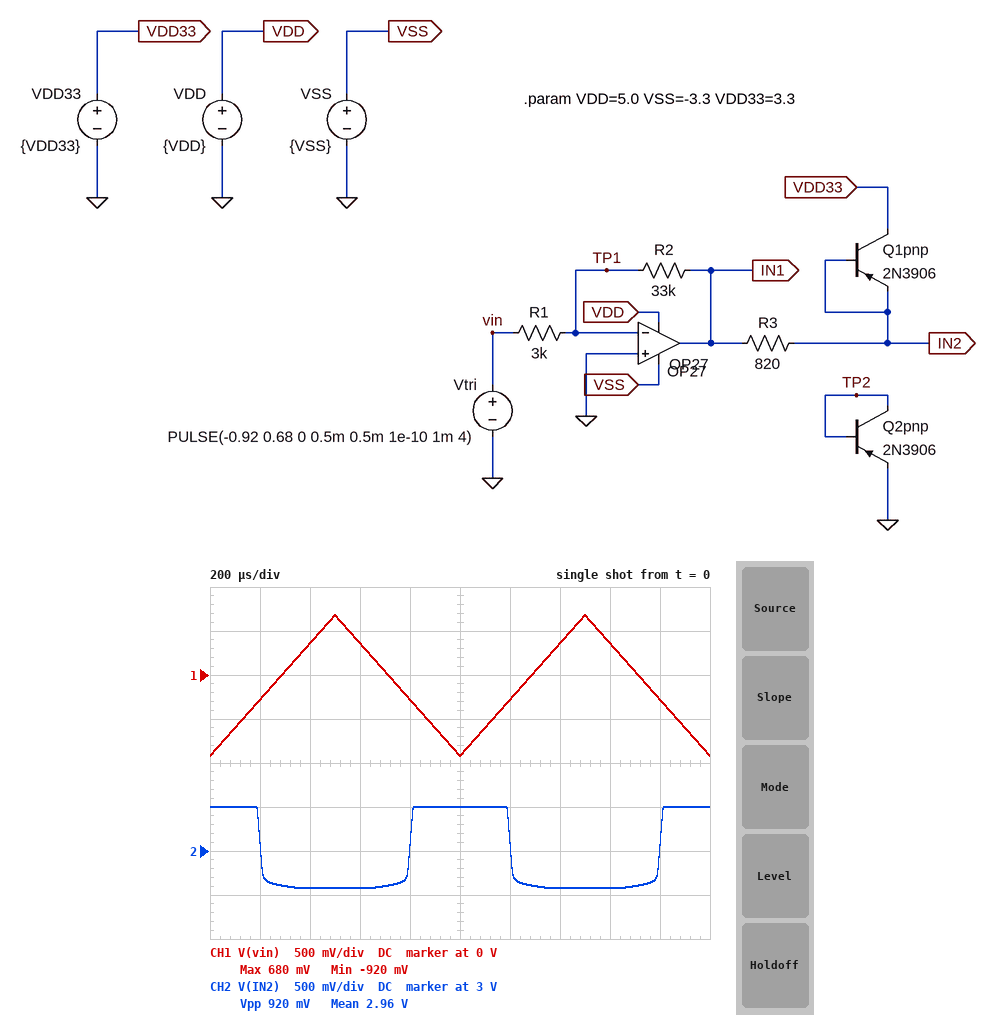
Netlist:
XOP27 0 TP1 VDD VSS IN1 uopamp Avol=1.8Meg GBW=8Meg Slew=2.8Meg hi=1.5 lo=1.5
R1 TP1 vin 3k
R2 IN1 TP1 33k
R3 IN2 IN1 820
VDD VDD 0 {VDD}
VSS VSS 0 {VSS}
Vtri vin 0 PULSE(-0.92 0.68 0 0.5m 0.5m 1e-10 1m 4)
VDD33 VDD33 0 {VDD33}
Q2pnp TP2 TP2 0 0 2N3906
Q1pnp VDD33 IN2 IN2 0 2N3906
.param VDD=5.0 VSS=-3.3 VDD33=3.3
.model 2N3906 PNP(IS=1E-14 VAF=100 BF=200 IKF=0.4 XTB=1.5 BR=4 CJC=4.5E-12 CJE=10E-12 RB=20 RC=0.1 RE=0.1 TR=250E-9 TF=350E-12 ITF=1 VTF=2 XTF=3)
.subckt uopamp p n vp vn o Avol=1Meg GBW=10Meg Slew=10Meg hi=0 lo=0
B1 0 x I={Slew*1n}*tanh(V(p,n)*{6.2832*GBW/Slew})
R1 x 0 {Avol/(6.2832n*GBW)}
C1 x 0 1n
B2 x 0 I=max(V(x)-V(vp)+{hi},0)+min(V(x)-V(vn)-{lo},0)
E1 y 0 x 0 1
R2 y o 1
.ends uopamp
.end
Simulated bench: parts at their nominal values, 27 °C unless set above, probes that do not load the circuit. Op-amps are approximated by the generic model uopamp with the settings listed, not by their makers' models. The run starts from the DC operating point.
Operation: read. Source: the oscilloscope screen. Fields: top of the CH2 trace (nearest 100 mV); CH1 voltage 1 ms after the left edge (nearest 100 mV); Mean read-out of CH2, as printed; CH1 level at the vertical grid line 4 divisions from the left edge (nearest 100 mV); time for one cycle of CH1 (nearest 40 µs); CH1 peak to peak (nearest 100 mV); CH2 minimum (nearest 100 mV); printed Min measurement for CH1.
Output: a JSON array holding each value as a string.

["3.5 V", "-900 mV", "2.96 V", "-300 mV", "1.00 ms", "1.6 V", "2.6 V", "-920 mV"]
